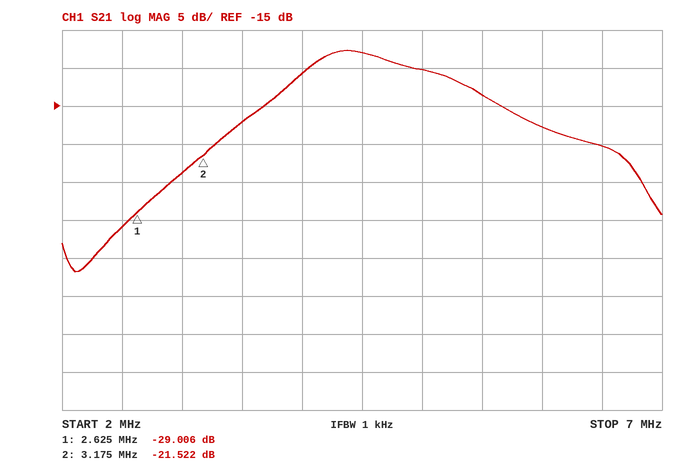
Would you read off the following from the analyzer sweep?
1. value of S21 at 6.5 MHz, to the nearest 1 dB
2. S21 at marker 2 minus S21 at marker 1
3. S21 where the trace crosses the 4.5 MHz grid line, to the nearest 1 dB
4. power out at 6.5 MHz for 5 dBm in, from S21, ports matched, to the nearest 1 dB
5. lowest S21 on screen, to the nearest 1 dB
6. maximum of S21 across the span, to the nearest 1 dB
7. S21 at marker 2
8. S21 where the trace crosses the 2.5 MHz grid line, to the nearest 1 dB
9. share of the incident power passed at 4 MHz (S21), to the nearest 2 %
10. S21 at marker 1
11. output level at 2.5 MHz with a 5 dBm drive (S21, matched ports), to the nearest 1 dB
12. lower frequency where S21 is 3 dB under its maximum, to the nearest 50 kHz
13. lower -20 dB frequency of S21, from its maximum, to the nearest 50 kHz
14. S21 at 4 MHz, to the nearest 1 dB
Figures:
-20 dB
7.484 dB
-8 dB
-15 dBm
-37 dB
-8 dB
-21.522 dB
-31 dB
8 %
-29.006 dB
-26 dBm
4.00 MHz
2.70 MHz
-11 dB
